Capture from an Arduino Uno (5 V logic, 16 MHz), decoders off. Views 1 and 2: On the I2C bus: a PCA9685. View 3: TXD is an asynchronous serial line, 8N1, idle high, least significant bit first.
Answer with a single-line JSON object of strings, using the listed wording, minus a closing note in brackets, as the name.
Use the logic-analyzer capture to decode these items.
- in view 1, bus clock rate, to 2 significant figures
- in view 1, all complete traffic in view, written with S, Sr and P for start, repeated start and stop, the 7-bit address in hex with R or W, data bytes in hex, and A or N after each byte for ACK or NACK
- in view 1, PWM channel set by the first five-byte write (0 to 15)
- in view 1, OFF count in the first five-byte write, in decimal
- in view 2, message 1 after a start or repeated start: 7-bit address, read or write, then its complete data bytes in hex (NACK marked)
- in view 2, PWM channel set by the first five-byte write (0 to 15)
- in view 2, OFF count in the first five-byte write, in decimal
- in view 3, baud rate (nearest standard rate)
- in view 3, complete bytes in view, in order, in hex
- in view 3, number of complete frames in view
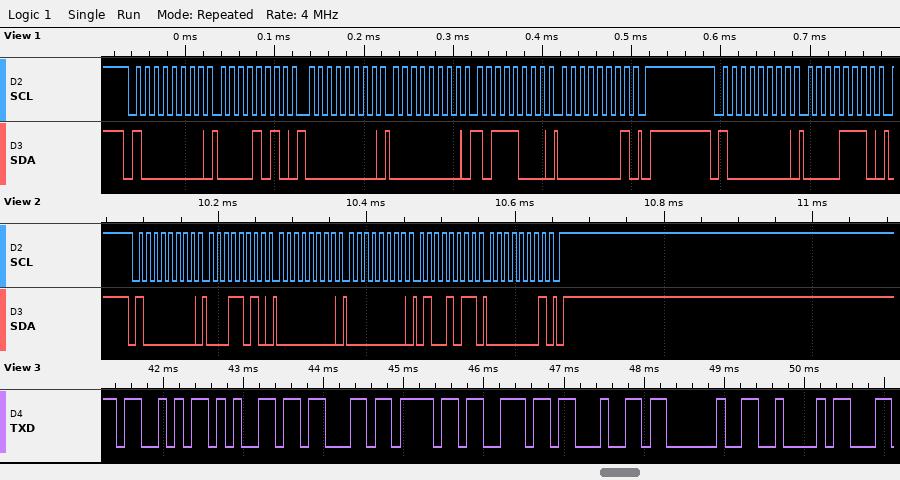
{"in view 1, bus clock rate, to 2 significant figures": "100 kHz", "in view 1, all complete traffic in view, written with S, Sr and P for start, repeated start and stop, the 7-bit address in hex with R or W, data bytes in hex, and A or N after each byte for ACK or NACK": "S 40W A 0A A 00 A 00 A B8 A 01 A P S 40W A 0E A", "in view 1, PWM channel set by the first five-byte write": "1", "in view 1, OFF count in the first five-byte write, in decimal": "440", "in view 2, message 1 after a start or repeated start: 7-bit address, read or write, then its complete data bytes in hex": "0x40 write: 1A 00 00 4B 01", "in view 2, PWM channel set by the first five-byte write": "5", "in view 2, OFF count in the first five-byte write, in decimal": "331", "in view 3, baud rate": "9600 baud", "in view 3, complete bytes in view, in order, in hex": "0x53 0x65 0x63 0x6F 0x6E 0x64 0x20 0x42", "in view 3, number of complete frames in view": "8"}
